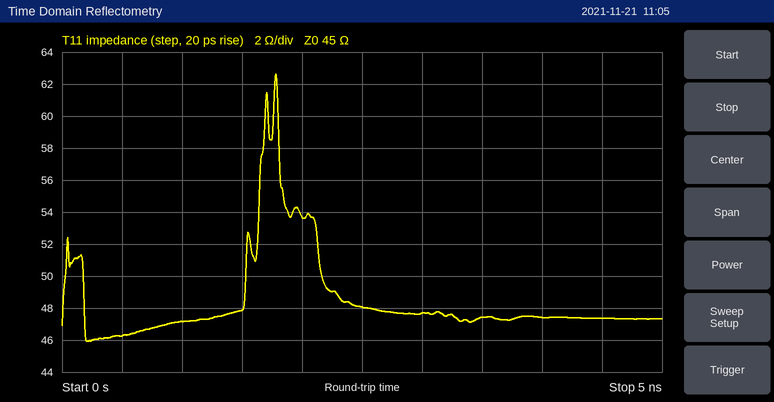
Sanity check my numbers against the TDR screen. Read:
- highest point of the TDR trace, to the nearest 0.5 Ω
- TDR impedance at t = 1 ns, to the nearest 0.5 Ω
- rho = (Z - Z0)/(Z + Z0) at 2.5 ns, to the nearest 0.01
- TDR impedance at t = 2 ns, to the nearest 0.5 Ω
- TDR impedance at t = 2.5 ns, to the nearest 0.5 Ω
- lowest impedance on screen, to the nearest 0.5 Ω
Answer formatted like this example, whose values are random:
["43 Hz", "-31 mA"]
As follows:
["62.5 Ω", "47.0 Ω", "+0.03", "53.5 Ω", "48.0 Ω", "46.0 Ω"]
